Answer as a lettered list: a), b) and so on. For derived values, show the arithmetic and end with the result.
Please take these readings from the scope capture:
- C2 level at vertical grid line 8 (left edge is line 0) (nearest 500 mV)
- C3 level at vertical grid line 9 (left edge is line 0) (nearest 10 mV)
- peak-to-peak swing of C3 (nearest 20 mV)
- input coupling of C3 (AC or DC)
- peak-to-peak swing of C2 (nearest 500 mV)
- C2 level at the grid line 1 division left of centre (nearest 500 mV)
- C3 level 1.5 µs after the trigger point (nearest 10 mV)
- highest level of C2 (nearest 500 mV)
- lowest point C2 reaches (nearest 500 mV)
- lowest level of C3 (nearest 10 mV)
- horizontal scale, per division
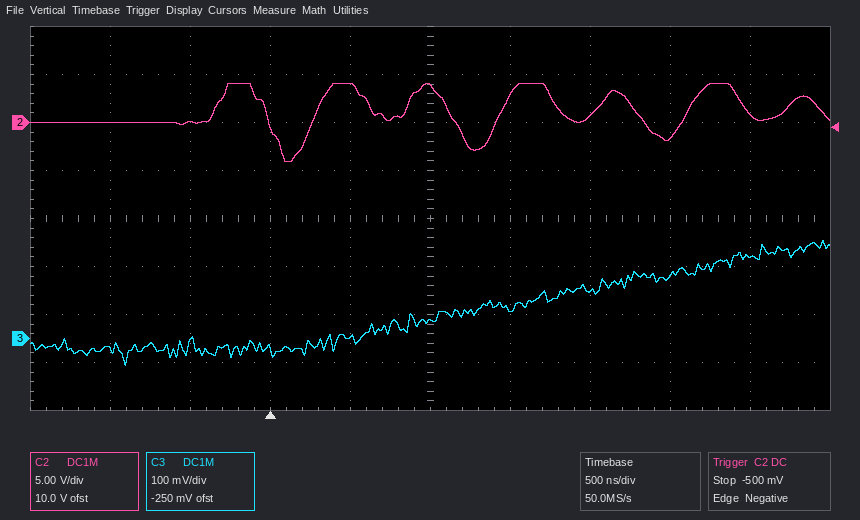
a) -1.5 V
b) 170 mV
c) 260 mV
d) DC
e) 4.0 V − (-4.0 V) = 8.0 V
f) 4.0 V
g) 60 mV
h) 4.0 V
i) -4.0 V
j) -60 mV
k) 500 ns
